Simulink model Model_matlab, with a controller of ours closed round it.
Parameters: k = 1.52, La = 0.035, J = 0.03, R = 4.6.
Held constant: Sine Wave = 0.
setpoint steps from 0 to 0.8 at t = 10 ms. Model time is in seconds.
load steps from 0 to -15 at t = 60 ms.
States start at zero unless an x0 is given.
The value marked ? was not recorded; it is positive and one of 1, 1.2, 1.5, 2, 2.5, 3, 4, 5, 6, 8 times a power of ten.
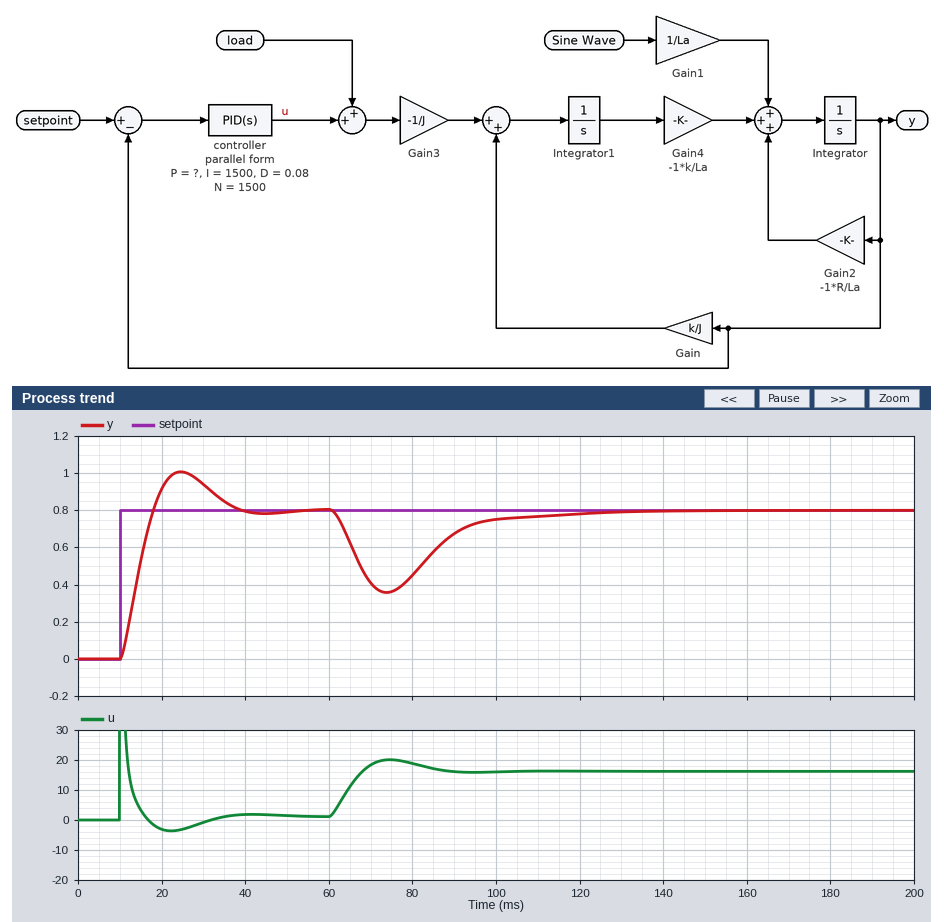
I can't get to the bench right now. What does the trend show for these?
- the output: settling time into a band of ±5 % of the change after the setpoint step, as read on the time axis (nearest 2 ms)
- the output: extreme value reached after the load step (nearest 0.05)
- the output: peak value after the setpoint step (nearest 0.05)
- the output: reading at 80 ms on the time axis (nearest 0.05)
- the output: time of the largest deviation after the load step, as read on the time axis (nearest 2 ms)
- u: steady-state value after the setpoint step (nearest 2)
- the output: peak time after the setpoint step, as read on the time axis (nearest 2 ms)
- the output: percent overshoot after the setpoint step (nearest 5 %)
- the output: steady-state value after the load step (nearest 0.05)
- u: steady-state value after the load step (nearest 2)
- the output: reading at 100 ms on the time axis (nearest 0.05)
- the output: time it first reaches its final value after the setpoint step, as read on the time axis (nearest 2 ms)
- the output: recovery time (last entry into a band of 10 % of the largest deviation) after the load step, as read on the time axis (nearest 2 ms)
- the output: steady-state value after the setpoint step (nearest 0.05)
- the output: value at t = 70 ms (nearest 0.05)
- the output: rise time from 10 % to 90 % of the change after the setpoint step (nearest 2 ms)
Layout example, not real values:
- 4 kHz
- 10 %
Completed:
- 36 ms
- 0.35
- 1.00
- 0.45
- 74 ms
- 2
- 24 ms
- 25 %
- 0.80
- 16
- 0.75
- 18 ms
- 102 ms
- 0.80
- 0.40
- 6 ms
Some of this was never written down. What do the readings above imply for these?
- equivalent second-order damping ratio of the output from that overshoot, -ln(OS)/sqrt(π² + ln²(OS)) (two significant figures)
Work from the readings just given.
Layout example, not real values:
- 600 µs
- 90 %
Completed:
- 0.40
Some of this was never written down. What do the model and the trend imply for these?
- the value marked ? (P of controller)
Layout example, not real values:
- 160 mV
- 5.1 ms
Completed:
- 30
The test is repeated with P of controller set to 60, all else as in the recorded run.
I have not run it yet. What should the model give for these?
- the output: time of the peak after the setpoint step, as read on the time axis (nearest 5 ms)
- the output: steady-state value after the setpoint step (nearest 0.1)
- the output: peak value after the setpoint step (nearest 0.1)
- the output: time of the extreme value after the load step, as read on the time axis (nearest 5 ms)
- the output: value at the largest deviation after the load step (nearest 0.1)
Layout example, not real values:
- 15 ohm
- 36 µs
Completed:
- 20 ms
- 0.8
- 1.1
- 70 ms
- 0.5
